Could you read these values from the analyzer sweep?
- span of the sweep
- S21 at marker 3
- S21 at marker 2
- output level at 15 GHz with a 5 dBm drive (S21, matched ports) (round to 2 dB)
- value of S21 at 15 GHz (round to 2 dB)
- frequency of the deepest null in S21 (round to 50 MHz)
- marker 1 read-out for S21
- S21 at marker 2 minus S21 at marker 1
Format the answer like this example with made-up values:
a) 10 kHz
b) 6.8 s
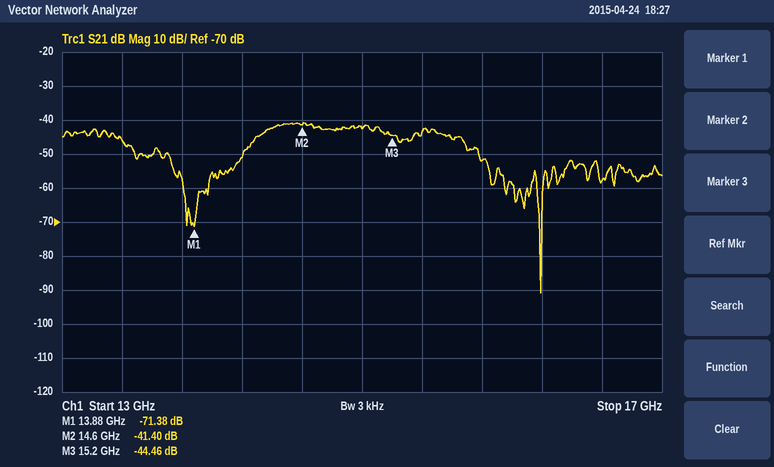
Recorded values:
a) 4 GHz
b) -44.46 dB
c) -41.40 dB
d) -38 dBm
e) -42 dB
f) 16.20 GHz
g) -71.38 dB
h) 29.98 dB
